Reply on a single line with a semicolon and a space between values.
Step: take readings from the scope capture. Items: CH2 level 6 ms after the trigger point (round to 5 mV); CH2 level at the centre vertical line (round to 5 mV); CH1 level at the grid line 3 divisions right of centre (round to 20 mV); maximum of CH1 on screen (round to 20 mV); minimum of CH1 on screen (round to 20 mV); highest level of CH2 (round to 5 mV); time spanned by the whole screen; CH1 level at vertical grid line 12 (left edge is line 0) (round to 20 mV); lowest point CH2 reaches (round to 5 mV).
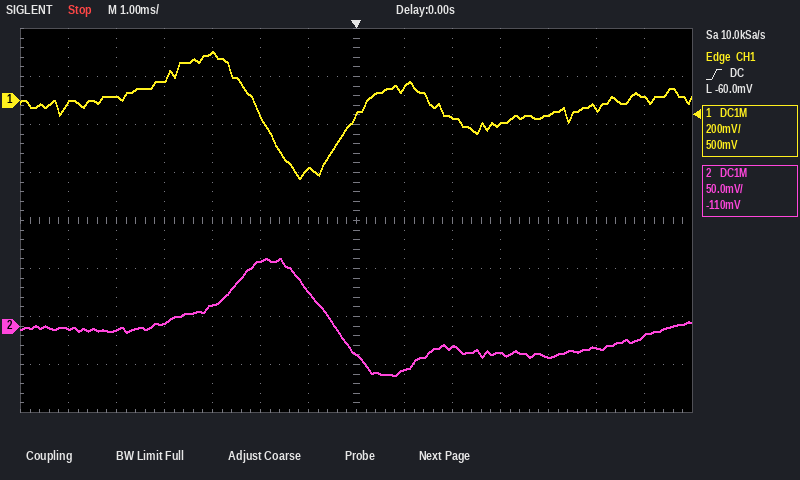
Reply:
-10 mV; -30 mV; -100 mV; 200 mV; -320 mV; 70 mV; 14 ms; -40 mV; -50 mV
